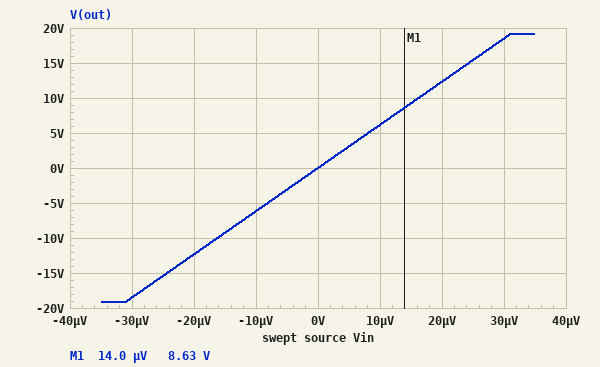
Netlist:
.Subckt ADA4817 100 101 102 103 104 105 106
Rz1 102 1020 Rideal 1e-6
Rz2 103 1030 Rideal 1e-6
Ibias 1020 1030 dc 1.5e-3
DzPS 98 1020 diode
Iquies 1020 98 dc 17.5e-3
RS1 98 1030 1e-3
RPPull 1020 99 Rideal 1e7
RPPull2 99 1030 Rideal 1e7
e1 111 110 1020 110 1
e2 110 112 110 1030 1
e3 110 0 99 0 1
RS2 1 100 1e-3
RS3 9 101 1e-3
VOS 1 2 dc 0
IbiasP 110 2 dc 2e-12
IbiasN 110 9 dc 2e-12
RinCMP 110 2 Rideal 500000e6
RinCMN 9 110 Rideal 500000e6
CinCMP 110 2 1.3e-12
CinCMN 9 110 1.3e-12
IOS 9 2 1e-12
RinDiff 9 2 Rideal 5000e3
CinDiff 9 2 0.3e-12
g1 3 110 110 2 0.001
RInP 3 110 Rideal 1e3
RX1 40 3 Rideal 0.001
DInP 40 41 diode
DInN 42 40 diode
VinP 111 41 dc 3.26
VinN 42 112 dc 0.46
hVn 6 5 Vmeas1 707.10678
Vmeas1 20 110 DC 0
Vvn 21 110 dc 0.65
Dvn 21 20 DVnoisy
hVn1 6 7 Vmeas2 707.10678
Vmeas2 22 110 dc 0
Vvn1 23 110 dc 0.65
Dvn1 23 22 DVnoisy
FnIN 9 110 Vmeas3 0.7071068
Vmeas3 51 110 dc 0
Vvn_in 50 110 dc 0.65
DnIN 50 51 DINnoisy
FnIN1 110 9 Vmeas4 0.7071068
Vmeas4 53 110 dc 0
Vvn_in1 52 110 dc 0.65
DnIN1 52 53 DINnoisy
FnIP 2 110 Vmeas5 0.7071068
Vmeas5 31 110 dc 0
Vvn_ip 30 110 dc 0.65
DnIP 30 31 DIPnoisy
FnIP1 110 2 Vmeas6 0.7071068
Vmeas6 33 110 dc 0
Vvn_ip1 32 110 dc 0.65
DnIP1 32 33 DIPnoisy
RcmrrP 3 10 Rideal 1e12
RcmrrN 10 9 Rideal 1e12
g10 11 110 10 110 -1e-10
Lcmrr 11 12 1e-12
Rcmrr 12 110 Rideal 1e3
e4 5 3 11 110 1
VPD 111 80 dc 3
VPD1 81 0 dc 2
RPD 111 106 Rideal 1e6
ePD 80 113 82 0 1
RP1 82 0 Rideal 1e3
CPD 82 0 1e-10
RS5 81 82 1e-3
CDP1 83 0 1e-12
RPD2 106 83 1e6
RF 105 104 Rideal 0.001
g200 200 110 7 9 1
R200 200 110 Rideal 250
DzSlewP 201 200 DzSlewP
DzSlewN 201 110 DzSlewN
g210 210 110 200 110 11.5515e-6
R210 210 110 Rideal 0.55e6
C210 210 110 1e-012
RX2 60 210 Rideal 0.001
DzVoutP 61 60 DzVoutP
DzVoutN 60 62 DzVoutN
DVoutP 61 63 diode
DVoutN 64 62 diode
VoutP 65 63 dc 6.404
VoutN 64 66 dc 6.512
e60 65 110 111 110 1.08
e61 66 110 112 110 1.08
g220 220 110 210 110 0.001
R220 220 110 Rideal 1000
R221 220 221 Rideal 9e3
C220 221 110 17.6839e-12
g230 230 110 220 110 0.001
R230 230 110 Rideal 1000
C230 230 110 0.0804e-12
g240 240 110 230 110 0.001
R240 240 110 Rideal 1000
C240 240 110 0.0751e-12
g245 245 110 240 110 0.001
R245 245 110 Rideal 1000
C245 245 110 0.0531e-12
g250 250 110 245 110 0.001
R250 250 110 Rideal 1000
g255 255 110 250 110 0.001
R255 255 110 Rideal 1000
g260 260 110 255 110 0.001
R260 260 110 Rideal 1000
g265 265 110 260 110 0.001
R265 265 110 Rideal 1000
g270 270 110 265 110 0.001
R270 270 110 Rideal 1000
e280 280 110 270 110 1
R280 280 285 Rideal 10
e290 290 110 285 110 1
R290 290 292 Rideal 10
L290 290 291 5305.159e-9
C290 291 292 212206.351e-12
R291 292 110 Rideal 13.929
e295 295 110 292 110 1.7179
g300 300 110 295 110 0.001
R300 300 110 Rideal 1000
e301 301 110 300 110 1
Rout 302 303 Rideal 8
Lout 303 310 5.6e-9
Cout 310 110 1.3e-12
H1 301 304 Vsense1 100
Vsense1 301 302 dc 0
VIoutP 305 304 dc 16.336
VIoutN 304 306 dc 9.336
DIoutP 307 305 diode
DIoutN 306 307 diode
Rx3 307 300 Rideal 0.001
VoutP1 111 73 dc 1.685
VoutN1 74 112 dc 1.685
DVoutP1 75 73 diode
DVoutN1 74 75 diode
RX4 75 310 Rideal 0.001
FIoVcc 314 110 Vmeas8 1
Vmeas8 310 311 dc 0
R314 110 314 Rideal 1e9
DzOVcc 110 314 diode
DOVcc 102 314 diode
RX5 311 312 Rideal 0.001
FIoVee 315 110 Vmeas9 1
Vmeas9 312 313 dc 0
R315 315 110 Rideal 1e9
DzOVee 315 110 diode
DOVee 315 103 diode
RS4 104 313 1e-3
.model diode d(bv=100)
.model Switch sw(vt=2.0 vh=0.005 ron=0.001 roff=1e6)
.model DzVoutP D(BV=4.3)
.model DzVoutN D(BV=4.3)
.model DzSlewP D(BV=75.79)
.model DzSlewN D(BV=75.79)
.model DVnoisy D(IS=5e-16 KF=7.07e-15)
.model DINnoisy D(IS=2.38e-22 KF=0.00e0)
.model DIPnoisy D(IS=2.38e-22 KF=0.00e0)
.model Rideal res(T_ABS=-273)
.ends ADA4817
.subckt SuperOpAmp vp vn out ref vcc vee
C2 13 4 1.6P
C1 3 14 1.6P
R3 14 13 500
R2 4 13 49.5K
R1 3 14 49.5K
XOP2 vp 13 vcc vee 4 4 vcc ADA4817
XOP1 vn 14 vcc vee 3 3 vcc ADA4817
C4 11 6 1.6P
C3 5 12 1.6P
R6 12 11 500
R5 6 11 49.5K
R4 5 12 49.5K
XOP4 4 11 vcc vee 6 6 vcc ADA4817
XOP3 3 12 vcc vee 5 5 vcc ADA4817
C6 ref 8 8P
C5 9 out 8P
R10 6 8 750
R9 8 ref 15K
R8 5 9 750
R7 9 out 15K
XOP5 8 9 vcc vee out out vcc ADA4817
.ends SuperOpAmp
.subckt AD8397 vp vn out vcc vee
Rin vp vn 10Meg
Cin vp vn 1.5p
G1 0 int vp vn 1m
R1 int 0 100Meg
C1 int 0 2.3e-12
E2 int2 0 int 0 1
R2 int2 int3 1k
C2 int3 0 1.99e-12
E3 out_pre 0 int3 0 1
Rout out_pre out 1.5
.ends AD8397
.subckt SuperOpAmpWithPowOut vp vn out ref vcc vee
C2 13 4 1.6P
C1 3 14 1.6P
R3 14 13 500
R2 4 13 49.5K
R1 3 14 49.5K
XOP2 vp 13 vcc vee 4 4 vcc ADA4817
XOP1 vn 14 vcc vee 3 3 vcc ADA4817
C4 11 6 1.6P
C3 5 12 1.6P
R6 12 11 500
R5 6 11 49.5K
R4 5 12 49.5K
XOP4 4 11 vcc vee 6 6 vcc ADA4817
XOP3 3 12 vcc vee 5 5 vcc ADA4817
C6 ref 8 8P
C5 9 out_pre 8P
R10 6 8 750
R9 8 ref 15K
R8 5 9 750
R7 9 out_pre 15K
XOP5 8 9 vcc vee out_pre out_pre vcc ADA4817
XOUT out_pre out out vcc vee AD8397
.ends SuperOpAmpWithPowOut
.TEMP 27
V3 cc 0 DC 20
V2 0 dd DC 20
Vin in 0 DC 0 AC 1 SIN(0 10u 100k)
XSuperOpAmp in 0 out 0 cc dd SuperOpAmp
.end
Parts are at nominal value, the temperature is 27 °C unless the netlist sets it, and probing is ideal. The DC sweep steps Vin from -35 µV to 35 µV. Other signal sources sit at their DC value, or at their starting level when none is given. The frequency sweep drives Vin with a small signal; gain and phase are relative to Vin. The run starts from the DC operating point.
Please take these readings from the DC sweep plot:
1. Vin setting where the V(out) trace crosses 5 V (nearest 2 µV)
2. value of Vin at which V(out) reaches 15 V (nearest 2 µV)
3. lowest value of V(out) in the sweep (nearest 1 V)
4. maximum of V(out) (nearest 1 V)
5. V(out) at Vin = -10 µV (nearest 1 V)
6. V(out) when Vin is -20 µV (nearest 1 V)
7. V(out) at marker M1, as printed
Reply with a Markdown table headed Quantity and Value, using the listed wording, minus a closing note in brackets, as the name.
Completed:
| Quantity | Value |
|---|---|
| Vin setting where the V(out) trace crosses 5 V | 8 µV |
| value of Vin at which V(out) reaches 15 V | 24 µV |
| lowest value of V(out) in the sweep | -19 V |
| maximum of V(out) | 19 V |
| V(out) at Vin = -10 µV | -6 V |
| V(out) when Vin is -20 µV | -12 V |
| V(out) at marker M1, as printed | 8.63 V |
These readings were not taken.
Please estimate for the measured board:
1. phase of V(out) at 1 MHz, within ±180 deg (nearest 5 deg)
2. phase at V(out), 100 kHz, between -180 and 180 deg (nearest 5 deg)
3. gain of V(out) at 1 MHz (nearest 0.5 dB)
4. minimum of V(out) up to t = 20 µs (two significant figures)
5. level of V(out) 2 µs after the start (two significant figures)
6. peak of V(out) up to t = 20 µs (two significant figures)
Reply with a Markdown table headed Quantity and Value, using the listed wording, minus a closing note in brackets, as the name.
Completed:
| Quantity | Value |
|---|---|
| phase of V(out) at 1 MHz, within ±180 deg | -125 deg |
| phase at V(out), 100 kHz, between -180 and 180 deg | -10 deg |
| gain of V(out) at 1 MHz | 109.5 dB |
| minimum of V(out) up to t = 20 µs | -6.6 V |
| level of V(out) 2 µs after the start | 5.6 V |
| peak of V(out) up to t = 20 µs | 6.6 V |
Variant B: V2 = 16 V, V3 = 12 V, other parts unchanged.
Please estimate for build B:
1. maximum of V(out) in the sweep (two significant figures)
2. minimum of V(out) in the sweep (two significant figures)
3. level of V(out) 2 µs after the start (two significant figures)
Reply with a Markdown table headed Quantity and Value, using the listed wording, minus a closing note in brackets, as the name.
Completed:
| Quantity | Value |
|---|---|
| maximum of V(out) in the sweep | 11 V |
| minimum of V(out) in the sweep | -15 V |
| level of V(out) 2 µs after the start | 5.6 V |
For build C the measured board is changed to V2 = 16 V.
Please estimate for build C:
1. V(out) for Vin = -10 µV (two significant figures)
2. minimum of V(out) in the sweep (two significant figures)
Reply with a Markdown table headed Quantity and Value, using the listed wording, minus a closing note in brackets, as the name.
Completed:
| Quantity | Value |
|---|---|
| V(out) for Vin = -10 µV | -6.1 V |
| minimum of V(out) in the sweep | -15 V |
